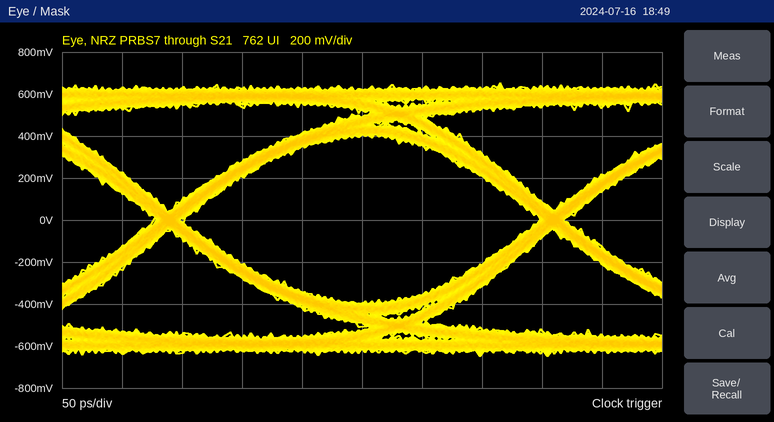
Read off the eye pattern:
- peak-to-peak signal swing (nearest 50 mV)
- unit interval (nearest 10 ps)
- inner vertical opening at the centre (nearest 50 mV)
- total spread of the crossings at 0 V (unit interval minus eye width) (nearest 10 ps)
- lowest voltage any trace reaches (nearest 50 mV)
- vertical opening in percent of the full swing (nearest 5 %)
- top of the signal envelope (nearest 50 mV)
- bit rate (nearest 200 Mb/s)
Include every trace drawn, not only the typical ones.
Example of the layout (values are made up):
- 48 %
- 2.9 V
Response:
- 1.30 V
- 320 ps
- 800 mV
- 20 ps
- -650 mV
- 60 %
- 650 mV
- 3.2 Gb/s
